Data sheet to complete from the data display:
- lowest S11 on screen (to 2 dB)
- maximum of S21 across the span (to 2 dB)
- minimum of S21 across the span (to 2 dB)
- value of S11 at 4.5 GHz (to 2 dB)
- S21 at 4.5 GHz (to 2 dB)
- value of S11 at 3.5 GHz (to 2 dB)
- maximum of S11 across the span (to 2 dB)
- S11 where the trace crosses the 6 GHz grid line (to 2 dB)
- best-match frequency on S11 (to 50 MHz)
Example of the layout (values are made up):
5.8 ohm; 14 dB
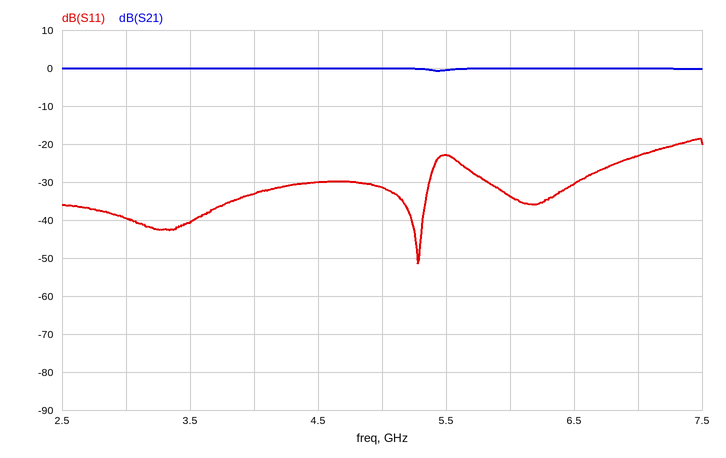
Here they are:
-52 dB; 0 dB; 0 dB; -30 dB; 0 dB; -40 dB; -18 dB; -34 dB; 5.30 GHz
